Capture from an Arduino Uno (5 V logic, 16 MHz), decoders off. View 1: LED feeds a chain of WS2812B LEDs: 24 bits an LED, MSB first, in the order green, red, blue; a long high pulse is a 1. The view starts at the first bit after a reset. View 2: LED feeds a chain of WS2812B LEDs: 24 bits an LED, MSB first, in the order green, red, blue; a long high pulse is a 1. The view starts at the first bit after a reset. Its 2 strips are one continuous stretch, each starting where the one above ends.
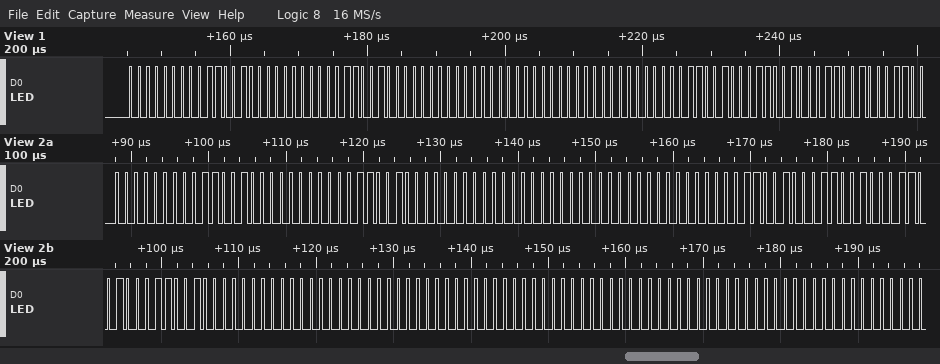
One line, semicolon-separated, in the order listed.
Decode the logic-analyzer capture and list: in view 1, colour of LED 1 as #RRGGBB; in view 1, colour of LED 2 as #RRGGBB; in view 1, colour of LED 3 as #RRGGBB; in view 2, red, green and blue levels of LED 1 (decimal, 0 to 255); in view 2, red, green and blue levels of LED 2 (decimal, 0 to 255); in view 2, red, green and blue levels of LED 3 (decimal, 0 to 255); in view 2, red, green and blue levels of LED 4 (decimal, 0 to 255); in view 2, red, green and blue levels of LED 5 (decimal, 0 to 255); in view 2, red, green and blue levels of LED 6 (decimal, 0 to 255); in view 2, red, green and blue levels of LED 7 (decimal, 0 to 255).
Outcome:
#640000; #006400; #000064; 100, 0, 0; 0, 100, 0; 0, 0, 100; 100, 100, 100; 0, 0, 0; 0, 0, 0; 0, 0, 0
